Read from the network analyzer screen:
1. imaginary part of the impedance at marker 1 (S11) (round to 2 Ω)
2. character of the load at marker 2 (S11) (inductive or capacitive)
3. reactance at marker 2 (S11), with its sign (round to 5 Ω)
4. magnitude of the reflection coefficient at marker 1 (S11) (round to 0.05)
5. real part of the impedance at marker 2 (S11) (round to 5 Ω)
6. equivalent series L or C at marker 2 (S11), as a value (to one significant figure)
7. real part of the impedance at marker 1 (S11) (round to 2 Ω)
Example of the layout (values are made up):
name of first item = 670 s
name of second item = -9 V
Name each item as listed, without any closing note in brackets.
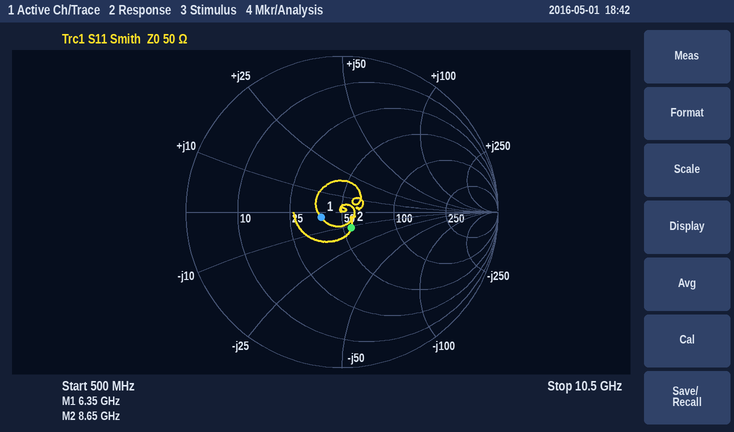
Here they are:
imaginary part of the impedance at marker 1 (S11) = -2 Ω
character of the load at marker 2 (S11) = capacitive
reactance at marker 2 (S11), with its sign = -10 Ω
magnitude of the reflection coefficient at marker 1 (S11) = 0.15
real part of the impedance at marker 2 (S11) = 55 Ω
equivalent series L or C at marker 2 (S11), as a value = 2 pF
real part of the impedance at marker 1 (S11) = 38 Ω
